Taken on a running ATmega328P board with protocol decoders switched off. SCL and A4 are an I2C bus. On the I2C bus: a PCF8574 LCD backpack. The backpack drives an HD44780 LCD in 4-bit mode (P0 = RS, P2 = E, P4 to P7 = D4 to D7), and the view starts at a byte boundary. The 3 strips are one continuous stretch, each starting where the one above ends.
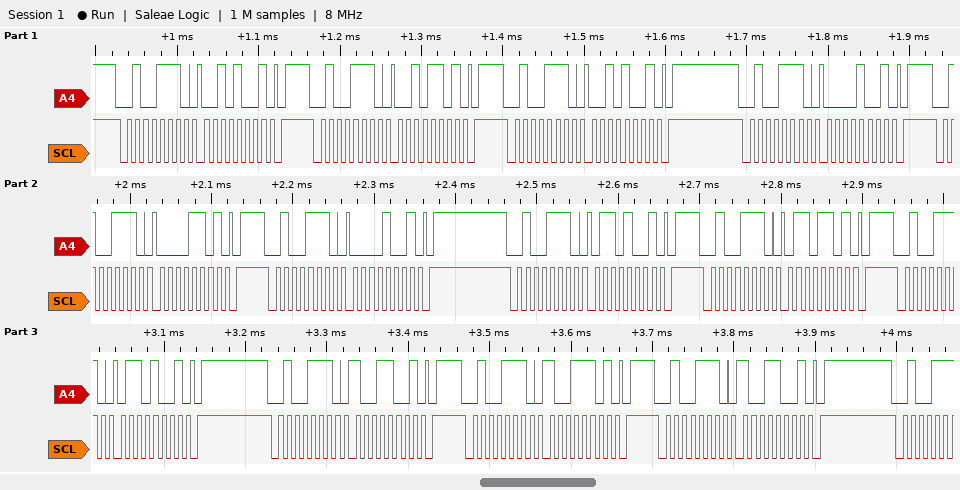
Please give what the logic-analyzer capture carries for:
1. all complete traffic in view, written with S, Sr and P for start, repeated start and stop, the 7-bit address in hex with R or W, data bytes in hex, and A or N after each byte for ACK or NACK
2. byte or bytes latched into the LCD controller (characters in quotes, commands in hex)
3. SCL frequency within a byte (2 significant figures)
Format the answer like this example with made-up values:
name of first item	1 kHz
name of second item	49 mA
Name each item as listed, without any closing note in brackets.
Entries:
all complete traffic in view, written with S, Sr and P for start, repeated start and stop, the 7-bit address in hex with R or W, data bytes in hex, and A or N after each byte for ACK or NACK	S 27W A 29 A P S 27W A 2D A P S 27W A 29 A P S 27W A 09 A P S 27W A 0D A P S 27W A 09 A P S 27W A 69 A P S 27W A 6D A P S 27W A 69 A P S 27W A 99 A P S 27W A 9D A P S 27W A 99 A P
byte or bytes latched into the LCD controller	' ' 'i'
SCL frequency within a byte	100 kHz
